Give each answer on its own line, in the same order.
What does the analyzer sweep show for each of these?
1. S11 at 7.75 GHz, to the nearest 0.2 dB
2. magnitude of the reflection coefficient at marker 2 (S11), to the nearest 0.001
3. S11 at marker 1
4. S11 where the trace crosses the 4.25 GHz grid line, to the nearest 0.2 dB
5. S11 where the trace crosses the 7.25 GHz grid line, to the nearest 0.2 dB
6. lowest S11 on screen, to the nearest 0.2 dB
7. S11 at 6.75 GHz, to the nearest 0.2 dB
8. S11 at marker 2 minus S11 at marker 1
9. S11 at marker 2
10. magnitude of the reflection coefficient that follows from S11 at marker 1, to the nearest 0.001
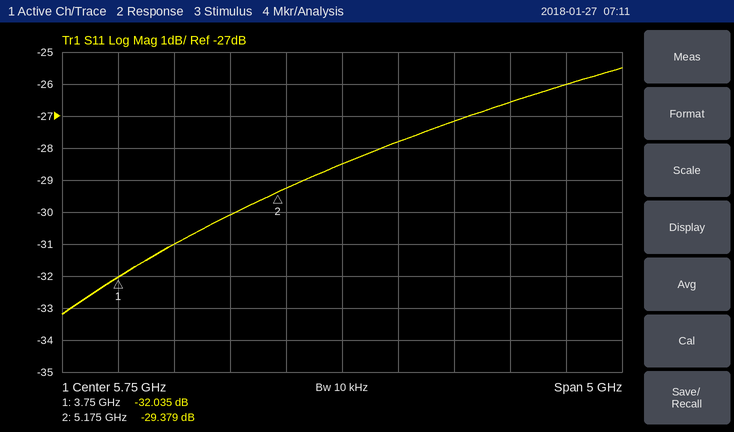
-26.0 dB
0.034
-32.035 dB
-31.0 dB
-26.6 dB
-33.2 dB
-27.2 dB
2.656 dB
-29.379 dB
0.025
